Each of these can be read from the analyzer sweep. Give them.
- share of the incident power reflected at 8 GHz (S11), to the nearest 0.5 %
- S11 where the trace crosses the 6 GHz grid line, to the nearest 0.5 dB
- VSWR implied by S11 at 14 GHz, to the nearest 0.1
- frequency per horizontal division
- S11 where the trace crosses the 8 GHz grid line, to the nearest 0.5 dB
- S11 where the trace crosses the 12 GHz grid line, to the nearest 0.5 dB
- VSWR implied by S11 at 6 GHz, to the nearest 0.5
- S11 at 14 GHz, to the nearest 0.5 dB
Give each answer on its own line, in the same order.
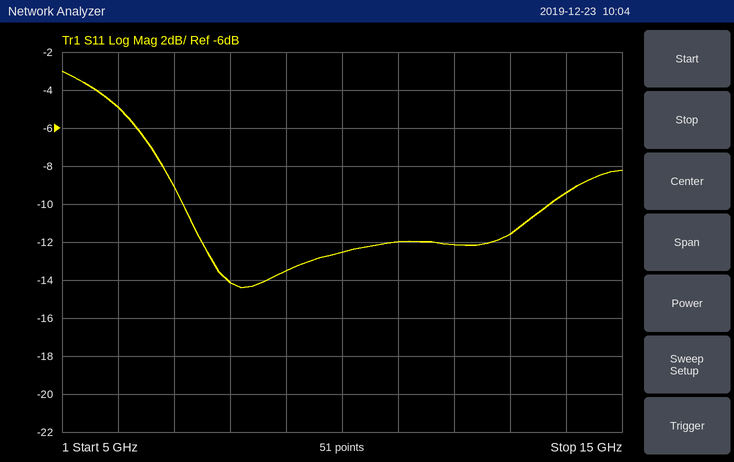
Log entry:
4.0 %
-5.0 dB
2.0
1 GHz
-14.0 dB
-12.0 dB
3.5
-9.5 dB
